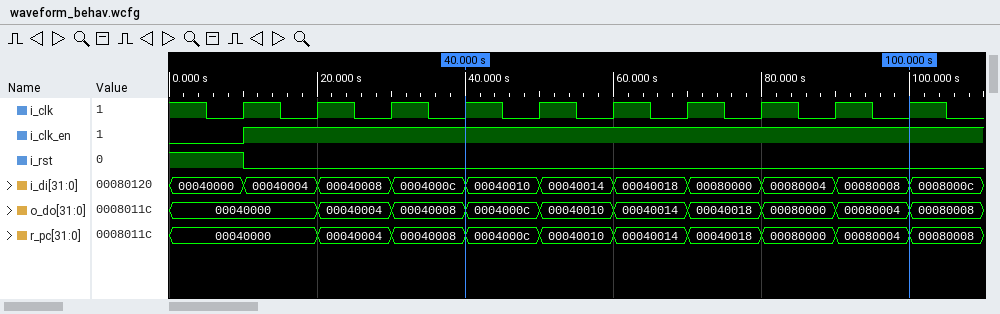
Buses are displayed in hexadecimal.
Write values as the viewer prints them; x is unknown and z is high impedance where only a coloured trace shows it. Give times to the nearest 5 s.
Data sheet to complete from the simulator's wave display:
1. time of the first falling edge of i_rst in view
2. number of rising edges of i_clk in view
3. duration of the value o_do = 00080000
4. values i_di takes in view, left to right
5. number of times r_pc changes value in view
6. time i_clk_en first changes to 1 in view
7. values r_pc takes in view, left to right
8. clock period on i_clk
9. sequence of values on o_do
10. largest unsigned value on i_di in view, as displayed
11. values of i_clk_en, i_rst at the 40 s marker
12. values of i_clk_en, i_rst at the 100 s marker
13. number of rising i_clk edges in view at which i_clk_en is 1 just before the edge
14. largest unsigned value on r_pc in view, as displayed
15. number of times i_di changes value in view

10 s
10
10 s
00040000, 00040004, 00040008, 0004000c, 00040010, 00040014, 00040018, 00080000, 00080004, 00080008, 0008000c
9
10 s
00040000, 00040004, 00040008, 0004000c, 00040010, 00040014, 00040018, 00080000, 00080004, 00080008
10 s
00040000, 00040004, 00040008, 0004000c, 00040010, 00040014, 00040018, 00080000, 00080004, 00080008
0008000c
i_clk_en=1, i_rst=0
i_clk_en=1, i_rst=0
9
00080008
10
